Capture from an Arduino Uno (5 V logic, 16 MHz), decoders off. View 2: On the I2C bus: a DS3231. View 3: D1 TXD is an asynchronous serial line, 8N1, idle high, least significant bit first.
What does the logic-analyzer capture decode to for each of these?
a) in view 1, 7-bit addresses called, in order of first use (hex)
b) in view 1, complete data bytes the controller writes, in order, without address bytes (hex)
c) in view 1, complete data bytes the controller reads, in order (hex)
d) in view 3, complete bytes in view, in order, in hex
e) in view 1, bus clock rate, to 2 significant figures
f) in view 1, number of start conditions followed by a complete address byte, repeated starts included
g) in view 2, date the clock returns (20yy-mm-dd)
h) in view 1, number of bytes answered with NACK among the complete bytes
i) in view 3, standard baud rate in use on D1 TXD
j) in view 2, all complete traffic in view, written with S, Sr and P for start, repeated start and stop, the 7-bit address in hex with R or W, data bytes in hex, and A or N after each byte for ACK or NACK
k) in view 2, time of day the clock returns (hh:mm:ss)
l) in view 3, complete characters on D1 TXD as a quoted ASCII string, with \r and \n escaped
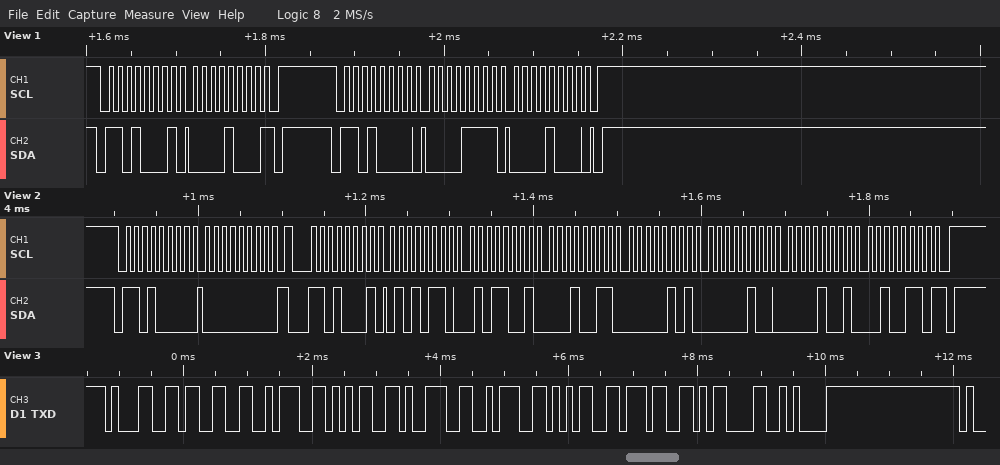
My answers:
0x68
0F 08
08
31 33 3A 35 39 3A 35 37 0D 0A
100 kHz
2
2026-09-04
1
9600 baud
S 68W A 00 A Sr 68R A 56 A 59 A 13 A 05 A 04 A 09 A 26 N P
13:59:56
"13:59:57\r\n"
